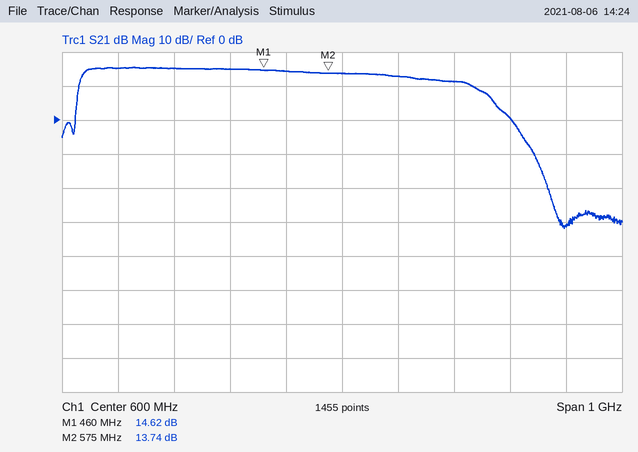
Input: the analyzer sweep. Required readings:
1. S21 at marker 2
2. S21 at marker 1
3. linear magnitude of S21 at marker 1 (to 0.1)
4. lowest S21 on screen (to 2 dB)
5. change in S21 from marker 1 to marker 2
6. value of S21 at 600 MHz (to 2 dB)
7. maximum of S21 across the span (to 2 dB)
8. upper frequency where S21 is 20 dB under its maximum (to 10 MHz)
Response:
13.74 dB
14.62 dB
5.4
-32 dB
-0.88 dB
14 dB
16 dB
920 MHz
